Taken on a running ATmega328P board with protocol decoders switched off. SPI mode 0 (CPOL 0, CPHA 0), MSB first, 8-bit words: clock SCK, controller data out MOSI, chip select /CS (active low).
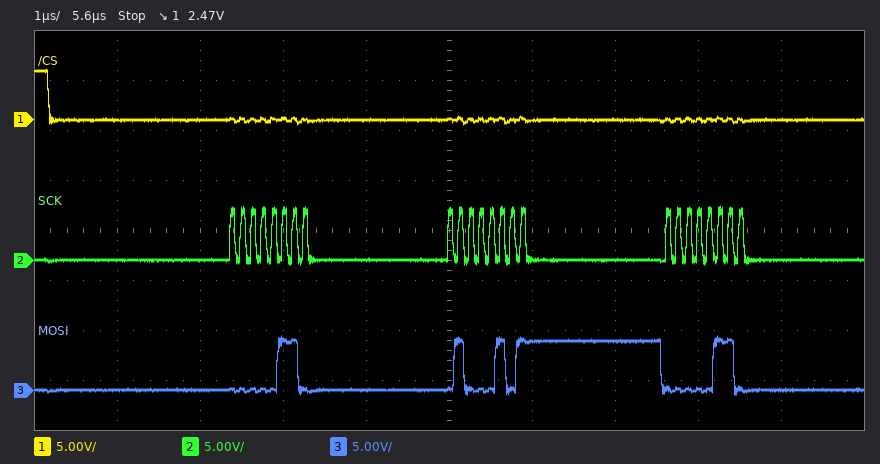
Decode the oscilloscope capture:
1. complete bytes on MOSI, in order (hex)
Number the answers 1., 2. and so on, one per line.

1. 06 45 06
